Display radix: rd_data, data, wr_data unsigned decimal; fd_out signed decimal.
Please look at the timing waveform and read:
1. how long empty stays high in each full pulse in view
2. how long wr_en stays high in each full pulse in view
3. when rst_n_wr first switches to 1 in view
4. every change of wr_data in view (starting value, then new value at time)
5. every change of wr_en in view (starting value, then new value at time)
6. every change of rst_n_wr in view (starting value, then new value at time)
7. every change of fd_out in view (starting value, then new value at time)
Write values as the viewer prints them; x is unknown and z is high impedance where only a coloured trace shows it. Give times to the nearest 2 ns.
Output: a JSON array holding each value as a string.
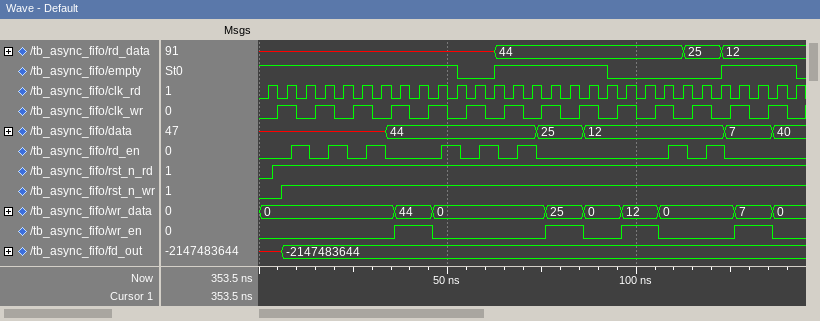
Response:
["30 ns, 20 ns", "10 ns, 10 ns, 10 ns, 10 ns", "6 ns", "0, 44 at 36 ns, 0 at 46 ns, 25 at 76 ns, 0 at 86 ns, 12 at 96 ns, 0 at 106 ns, 7 at 126 ns, 0 at 136 ns", "0, 1 at 36 ns, 0 at 46 ns, 1 at 76 ns, 0 at 86 ns, 1 at 96 ns, 0 at 106 ns, 1 at 126 ns, 0 at 136 ns", "0, 1 at 6 ns", "x, -2147483644 at 6 ns"]
